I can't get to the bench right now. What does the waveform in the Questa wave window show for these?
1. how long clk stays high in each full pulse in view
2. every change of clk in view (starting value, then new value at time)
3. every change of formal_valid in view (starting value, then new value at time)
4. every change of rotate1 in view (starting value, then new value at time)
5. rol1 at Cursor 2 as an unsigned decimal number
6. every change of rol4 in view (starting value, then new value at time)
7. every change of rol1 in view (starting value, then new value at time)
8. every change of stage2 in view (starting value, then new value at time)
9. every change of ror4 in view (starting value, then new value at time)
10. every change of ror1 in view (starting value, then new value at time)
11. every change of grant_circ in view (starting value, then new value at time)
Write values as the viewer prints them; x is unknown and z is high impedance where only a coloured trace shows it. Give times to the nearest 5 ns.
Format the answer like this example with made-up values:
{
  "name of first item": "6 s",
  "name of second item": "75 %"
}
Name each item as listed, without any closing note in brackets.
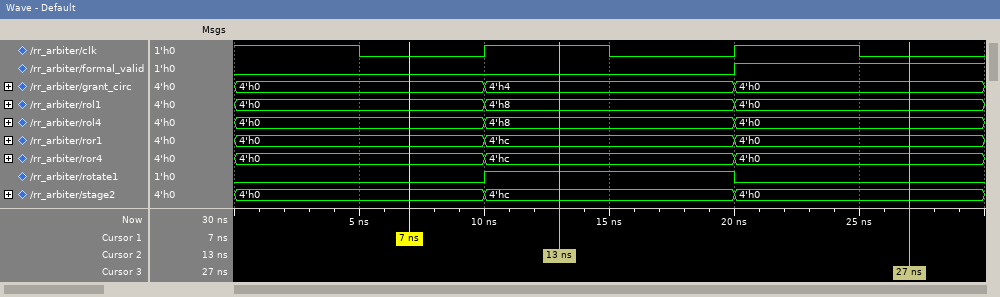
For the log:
{
  "how long clk stays high in each full pulse in view": "5 ns, 5 ns",
  "every change of clk in view": "1, 0 at 5 ns, 1 at 10 ns, 0 at 15 ns, 1 at 20 ns, 0 at 25 ns",
  "every change of formal_valid in view": "0, 1 at 20 ns",
  "every change of rotate1 in view": "0, 1 at 10 ns, 0 at 20 ns",
  "rol1 at Cursor 2 as an unsigned decimal number": "8",
  "every change of rol4 in view": "4'h0, 4'h8 at 10 ns, 4'h0 at 20 ns",
  "every change of rol1 in view": "4'h0, 4'h8 at 10 ns, 4'h0 at 20 ns",
  "every change of stage2 in view": "4'h0, 4'hc at 10 ns, 4'h0 at 20 ns",
  "every change of ror4 in view": "4'h0, 4'hc at 10 ns, 4'h0 at 20 ns",
  "every change of ror1 in view": "4'h0, 4'hc at 10 ns, 4'h0 at 20 ns",
  "every change of grant_circ in view": "4'h0, 4'h4 at 10 ns, 4'h0 at 20 ns"
}
